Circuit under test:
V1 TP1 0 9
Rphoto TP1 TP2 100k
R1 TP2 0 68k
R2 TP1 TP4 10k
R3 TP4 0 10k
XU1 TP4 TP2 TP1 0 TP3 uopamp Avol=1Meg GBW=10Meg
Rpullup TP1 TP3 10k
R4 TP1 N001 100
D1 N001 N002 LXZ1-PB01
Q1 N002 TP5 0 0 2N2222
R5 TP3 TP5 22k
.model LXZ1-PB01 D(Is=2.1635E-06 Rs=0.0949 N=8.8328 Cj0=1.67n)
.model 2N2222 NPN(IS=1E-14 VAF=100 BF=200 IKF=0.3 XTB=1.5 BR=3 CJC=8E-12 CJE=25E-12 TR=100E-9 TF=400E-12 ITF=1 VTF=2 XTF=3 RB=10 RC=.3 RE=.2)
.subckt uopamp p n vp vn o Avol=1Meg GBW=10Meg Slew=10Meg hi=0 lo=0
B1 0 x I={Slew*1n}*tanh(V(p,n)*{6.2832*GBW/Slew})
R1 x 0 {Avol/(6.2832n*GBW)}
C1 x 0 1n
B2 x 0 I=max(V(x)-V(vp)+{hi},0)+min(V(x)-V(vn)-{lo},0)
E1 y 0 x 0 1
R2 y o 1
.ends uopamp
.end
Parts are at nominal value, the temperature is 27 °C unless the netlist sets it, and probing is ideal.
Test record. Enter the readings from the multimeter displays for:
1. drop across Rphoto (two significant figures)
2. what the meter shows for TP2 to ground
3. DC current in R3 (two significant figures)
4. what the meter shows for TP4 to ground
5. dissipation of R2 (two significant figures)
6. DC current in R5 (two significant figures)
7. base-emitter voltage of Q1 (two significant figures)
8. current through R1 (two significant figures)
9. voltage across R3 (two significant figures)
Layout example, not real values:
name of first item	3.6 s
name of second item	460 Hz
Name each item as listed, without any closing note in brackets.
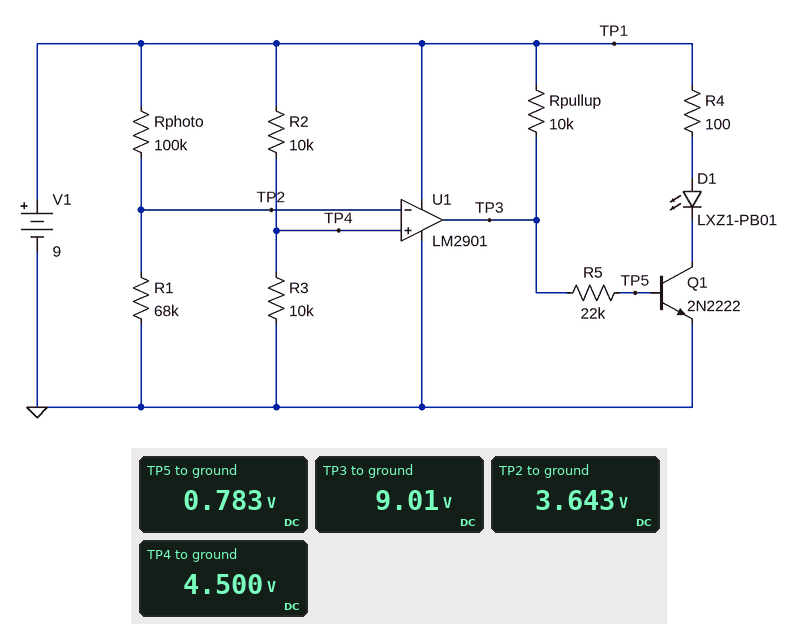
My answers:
drop across Rphoto	5.4 V
what the meter shows for TP2 to ground	3.643 V
DC current in R3	450 µA
what the meter shows for TP4 to ground	4.500 V
dissipation of R2	2.0 mW
DC current in R5	370 µA
base-emitter voltage of Q1	780 mV
current through R1	54 µA
voltage across R3	4.5 V
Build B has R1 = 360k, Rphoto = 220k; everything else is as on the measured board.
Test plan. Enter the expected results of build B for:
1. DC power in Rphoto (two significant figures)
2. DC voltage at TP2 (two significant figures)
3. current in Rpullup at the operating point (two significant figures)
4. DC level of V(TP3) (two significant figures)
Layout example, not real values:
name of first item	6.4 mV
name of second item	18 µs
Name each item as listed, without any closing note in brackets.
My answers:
DC power in Rphoto	53 µW
DC voltage at TP2	5.6 V
current in Rpullup at the operating point	900 µA
DC level of V(TP3)	-9.1 mV
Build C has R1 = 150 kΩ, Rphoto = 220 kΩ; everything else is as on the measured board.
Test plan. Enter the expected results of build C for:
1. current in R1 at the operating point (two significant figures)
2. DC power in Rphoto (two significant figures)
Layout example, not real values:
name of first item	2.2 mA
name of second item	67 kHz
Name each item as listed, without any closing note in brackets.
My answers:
current in R1 at the operating point	24 µA
DC power in Rphoto	130 µW
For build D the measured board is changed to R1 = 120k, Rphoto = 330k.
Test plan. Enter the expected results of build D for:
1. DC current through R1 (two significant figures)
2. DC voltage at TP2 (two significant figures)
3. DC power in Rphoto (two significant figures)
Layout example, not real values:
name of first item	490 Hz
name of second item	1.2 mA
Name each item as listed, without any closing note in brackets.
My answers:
DC current through R1	20 µA
DC voltage at TP2	2.4 V
DC power in Rphoto	130 µW
